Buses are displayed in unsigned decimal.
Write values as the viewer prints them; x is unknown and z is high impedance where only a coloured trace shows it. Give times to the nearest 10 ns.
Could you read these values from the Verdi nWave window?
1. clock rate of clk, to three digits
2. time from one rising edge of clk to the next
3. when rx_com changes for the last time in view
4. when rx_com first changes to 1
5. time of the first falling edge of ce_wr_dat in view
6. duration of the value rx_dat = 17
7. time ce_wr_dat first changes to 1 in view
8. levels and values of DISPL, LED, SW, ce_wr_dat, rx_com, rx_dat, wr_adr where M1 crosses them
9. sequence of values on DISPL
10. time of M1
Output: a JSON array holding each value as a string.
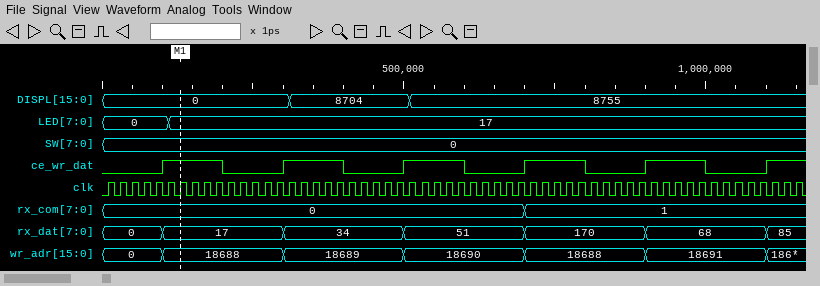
["50.0 MHz", "20 ns", "700 ns", "700 ns", "200 ns", "200 ns", "100 ns", "DISPL=0, LED=17, SW=0, ce_wr_dat=1, rx_com=0, rx_dat=17, wr_adr=18688", "0, 8704, 8755", "130 ns"]
